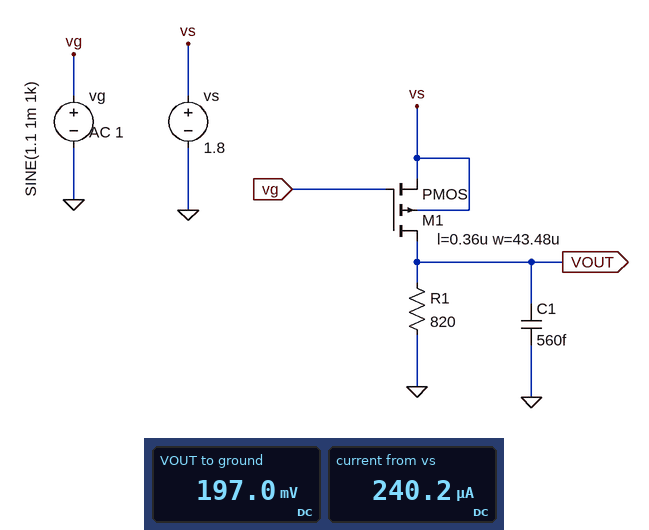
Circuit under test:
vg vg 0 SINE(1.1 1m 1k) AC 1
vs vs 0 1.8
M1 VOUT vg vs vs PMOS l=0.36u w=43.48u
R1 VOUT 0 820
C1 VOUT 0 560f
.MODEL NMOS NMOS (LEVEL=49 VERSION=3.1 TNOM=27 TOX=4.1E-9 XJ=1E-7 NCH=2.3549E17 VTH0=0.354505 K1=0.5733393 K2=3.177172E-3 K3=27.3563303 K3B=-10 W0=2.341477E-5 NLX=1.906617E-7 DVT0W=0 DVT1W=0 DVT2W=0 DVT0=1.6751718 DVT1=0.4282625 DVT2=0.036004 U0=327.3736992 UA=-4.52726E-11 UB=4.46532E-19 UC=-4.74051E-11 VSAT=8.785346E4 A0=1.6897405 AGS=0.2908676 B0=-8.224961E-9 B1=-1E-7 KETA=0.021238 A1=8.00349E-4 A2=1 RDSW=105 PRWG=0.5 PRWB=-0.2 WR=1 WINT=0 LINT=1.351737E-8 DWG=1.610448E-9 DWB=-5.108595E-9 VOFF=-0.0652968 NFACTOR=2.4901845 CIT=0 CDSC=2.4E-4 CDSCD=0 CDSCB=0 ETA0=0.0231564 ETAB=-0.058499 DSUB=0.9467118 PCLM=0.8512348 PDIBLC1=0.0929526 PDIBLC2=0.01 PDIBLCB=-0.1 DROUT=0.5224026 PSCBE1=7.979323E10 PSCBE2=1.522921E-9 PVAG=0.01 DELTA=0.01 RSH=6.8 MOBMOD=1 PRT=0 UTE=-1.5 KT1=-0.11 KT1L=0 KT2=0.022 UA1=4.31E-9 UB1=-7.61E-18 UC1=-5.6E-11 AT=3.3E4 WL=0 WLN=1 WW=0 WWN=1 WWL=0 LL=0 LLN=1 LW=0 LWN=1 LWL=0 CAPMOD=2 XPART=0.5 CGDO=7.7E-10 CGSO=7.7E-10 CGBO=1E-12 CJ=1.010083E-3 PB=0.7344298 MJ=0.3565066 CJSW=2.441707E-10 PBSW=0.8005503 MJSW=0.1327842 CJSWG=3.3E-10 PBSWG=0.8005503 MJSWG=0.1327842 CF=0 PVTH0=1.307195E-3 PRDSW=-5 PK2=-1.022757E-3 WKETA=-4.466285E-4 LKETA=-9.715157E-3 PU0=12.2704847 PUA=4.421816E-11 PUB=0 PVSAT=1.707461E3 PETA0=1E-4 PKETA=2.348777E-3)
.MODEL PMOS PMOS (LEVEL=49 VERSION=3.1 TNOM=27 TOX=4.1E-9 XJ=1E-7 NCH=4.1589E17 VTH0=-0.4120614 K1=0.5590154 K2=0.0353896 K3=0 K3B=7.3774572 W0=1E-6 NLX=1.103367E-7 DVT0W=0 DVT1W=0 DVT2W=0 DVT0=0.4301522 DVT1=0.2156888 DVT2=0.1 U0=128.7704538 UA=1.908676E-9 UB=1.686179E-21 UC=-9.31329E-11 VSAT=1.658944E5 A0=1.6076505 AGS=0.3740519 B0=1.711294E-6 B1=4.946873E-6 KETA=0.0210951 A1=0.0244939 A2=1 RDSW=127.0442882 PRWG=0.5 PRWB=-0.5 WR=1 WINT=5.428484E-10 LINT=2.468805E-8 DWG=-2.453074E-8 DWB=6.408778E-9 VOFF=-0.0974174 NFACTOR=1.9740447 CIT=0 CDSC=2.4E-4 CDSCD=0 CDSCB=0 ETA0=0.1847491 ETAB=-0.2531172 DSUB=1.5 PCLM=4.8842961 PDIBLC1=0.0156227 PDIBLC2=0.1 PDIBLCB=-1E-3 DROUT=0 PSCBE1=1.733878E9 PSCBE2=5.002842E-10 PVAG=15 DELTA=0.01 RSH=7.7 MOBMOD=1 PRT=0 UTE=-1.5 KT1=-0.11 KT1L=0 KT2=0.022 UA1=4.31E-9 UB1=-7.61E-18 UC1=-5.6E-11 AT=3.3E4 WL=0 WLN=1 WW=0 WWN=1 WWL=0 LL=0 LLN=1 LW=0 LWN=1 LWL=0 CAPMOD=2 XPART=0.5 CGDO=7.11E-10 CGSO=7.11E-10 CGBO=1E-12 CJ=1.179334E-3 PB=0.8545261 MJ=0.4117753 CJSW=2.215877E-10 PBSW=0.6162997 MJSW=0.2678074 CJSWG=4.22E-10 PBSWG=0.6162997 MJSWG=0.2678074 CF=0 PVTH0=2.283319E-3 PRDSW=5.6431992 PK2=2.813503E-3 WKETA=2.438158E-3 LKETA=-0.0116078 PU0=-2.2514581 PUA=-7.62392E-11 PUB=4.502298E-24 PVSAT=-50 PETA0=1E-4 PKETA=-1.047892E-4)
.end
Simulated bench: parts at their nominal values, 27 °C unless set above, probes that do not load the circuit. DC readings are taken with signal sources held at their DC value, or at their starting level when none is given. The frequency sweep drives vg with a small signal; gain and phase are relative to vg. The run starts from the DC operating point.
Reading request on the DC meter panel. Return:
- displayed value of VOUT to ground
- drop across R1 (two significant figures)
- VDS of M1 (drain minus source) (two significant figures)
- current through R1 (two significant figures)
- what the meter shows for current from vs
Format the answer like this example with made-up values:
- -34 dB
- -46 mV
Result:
- 197.0 mV
- 200 mV
- -1.6 V
- 240 µA
- 240.2 µA
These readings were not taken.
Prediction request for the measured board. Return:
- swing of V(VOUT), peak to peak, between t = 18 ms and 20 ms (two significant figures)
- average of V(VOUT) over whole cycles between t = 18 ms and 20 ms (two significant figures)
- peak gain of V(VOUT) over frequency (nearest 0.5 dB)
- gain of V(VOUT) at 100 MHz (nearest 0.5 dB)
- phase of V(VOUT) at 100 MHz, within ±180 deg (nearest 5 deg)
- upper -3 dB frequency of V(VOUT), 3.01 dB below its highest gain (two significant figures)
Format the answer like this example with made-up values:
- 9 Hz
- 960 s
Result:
- 3.1 mV
- 200 mV
- 4.0 dB
- 3.5 dB
- 160 deg
- 330 MHz
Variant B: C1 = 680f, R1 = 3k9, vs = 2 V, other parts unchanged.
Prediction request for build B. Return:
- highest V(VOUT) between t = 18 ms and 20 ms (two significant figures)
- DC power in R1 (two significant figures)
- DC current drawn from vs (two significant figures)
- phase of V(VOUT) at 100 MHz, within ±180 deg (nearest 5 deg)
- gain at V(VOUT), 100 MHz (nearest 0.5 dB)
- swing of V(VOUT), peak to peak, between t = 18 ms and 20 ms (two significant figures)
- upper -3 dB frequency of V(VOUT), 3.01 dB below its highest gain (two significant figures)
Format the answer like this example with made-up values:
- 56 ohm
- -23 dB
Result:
- 1.8 V
- 860 µW
- 470 µA
- 165 deg
- -4.5 dB
- 1.2 mV
- 470 MHz
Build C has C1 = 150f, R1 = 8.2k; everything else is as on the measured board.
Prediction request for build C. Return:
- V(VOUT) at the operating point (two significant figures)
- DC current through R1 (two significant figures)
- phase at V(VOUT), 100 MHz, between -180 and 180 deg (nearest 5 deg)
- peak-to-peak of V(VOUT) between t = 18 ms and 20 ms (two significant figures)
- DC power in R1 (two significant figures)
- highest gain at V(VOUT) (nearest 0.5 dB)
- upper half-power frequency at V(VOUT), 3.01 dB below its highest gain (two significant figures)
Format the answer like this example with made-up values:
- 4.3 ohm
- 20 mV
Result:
- 1.6 V
- 200 µA
- 165 deg
- 6.1 mV
- 320 µW
- 9.5 dB
- 370 MHz
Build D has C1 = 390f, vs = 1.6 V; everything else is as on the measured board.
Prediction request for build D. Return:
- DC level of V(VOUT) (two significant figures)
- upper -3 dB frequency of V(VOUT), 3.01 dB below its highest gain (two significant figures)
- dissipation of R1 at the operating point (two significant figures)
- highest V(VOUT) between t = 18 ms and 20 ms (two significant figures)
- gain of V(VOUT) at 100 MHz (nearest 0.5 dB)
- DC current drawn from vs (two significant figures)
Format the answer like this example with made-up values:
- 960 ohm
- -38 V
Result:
- 13 mV
- 620 MHz
- 220 nW
- 14 mV
- -11.5 dB
- 16 µA
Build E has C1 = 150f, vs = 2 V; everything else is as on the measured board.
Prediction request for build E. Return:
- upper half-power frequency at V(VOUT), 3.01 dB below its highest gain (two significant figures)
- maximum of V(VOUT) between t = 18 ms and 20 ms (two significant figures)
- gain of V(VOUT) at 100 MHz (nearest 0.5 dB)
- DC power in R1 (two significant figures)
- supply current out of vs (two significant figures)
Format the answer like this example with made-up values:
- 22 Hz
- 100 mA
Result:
- 1.1 GHz
- 600 mV
- 7.5 dB
- 440 µW
- 730 µA
